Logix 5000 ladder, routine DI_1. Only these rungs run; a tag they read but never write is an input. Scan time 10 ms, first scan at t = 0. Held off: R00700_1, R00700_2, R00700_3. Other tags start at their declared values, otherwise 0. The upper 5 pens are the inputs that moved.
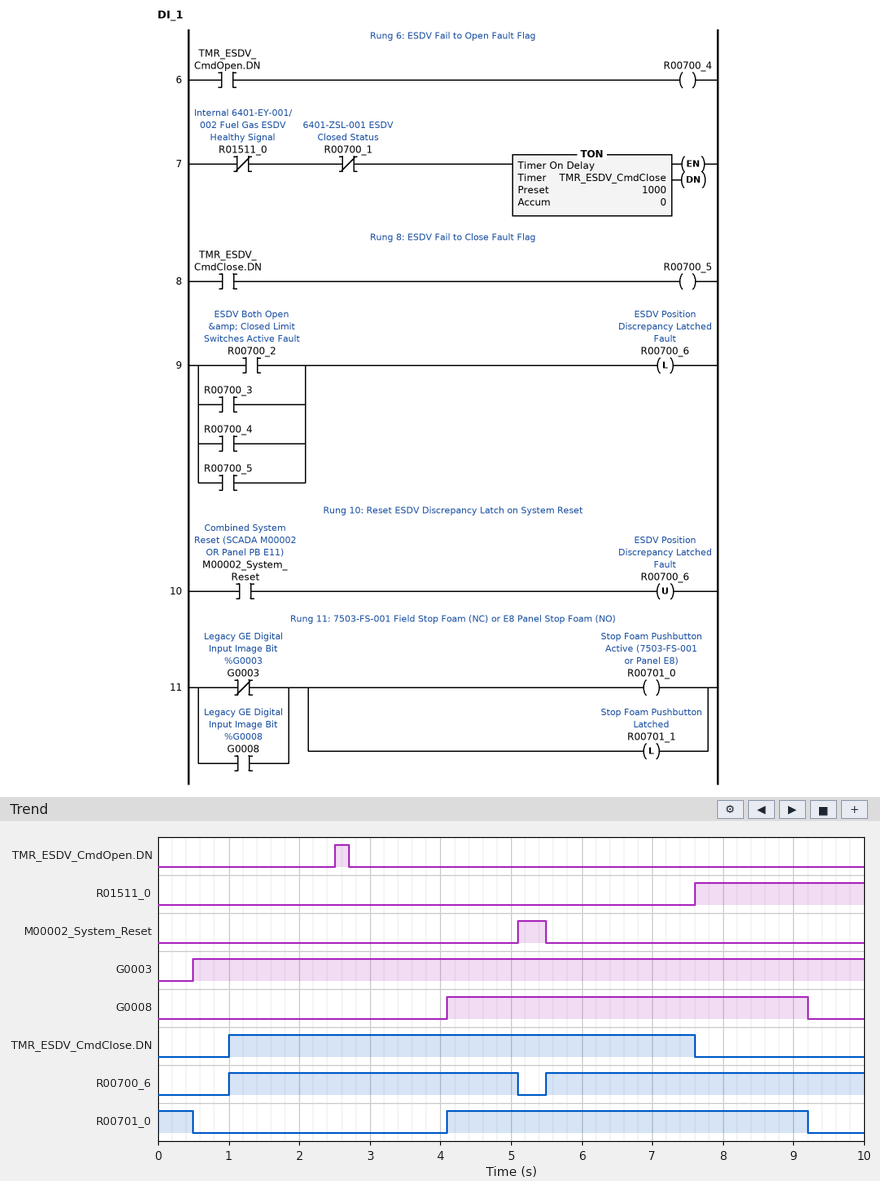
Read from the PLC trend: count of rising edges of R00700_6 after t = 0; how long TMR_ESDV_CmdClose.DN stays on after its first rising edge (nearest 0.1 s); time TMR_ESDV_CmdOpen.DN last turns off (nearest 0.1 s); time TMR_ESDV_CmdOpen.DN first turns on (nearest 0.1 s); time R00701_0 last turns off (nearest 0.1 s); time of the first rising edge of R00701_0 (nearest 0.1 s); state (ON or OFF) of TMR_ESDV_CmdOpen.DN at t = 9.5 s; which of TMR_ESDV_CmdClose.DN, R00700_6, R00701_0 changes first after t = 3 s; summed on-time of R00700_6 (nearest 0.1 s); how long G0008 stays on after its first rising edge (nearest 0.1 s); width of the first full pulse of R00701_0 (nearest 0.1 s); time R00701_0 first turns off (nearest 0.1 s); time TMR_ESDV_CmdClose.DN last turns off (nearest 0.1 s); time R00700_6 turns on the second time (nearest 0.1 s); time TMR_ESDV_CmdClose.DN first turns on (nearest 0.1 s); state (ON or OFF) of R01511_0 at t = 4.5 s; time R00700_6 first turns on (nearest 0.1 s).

2
6.6 s
2.7 s
2.5 s
9.2 s
4.1 s
OFF
R00701_0
8.6 s
5.1 s
5.1 s
0.5 s
7.6 s
5.5 s
1.0 s
OFF
1.0 s
